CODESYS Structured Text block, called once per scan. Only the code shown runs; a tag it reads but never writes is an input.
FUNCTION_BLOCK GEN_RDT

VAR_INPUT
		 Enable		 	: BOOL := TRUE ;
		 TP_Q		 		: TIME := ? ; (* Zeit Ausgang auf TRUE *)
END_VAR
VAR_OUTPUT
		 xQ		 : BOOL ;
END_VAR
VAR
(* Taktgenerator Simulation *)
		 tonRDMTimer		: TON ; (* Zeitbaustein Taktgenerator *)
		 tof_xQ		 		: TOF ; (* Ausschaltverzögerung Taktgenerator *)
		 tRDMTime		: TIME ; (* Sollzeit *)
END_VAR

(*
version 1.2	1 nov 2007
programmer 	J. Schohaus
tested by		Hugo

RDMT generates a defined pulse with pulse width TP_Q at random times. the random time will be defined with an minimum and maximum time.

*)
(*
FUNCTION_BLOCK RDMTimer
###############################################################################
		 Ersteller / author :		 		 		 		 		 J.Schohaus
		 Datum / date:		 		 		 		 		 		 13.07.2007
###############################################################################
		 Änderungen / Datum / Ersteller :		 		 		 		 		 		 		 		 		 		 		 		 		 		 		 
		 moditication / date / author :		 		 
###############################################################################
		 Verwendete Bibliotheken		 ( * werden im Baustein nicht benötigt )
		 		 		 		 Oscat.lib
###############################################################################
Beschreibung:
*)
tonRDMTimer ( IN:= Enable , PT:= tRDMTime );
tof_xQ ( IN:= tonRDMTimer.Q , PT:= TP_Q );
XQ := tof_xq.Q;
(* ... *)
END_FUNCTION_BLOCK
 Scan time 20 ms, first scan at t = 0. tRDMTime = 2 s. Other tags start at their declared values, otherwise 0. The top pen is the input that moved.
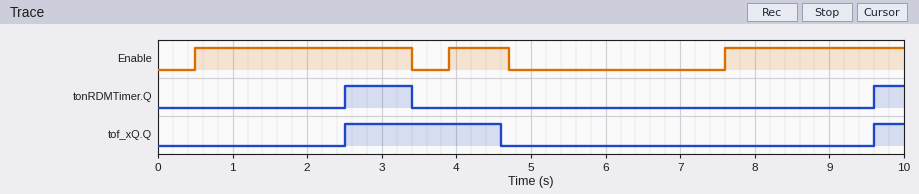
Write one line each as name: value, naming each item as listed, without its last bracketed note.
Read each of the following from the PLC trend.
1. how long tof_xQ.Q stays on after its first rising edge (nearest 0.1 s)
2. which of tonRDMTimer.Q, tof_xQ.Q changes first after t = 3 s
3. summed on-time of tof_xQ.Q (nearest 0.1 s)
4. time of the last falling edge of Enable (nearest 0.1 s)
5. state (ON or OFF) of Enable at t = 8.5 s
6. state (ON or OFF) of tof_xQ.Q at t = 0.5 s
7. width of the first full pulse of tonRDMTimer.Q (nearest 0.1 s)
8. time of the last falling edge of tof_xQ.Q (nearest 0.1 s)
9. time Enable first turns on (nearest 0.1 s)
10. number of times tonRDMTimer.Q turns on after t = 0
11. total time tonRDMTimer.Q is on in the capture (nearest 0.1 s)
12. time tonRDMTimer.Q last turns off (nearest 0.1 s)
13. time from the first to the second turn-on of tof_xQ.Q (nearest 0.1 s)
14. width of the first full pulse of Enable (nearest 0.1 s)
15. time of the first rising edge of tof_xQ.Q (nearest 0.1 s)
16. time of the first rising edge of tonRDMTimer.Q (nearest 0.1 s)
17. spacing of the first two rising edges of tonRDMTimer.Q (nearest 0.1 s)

how long tof_xQ.Q stays on after its first rising edge: 2.1 s
which of tonRDMTimer.Q, tof_xQ.Q changes first after t = 3 s: tonRDMTimer.Q
summed on-time of tof_xQ.Q: 2.5 s
time of the last falling edge of Enable: 4.7 s
state (ON or OFF) of Enable at t = 8.5 s: ON
state (ON or OFF) of tof_xQ.Q at t = 0.5 s: OFF
width of the first full pulse of tonRDMTimer.Q: 0.9 s
time of the last falling edge of tof_xQ.Q: 4.6 s
time Enable first turns on: 0.5 s
number of times tonRDMTimer.Q turns on after t = 0: 2
total time tonRDMTimer.Q is on in the capture: 1.3 s
time tonRDMTimer.Q last turns off: 3.4 s
time from the first to the second turn-on of tof_xQ.Q: 7.1 s
width of the first full pulse of Enable: 2.9 s
time of the first rising edge of tof_xQ.Q: 2.5 s
time of the first rising edge of tonRDMTimer.Q: 2.5 s
spacing of the first two rising edges of tonRDMTimer.Q: 7.1 s
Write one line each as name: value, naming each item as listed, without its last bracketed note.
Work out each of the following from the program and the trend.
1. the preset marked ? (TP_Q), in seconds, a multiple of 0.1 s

the preset marked ? (TP_Q), in seconds, a multiple of 0.1 s: 1.2 s
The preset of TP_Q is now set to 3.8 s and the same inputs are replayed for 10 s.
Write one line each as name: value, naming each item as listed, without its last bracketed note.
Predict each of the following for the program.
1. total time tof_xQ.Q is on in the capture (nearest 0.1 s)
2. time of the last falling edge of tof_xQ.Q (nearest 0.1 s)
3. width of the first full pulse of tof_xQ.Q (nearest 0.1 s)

total time tof_xQ.Q is on in the capture: 5.1 s
time of the last falling edge of tof_xQ.Q: 7.2 s
width of the first full pulse of tof_xQ.Q: 4.7 s
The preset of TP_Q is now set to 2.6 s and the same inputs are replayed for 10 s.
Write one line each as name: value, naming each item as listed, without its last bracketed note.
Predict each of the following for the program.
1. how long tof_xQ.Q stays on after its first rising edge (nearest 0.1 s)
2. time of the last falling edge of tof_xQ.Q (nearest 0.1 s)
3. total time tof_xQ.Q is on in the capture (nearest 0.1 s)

how long tof_xQ.Q stays on after its first rising edge: 3.5 s
time of the last falling edge of tof_xQ.Q: 6.0 s
total time tof_xQ.Q is on in the capture: 3.9 s
